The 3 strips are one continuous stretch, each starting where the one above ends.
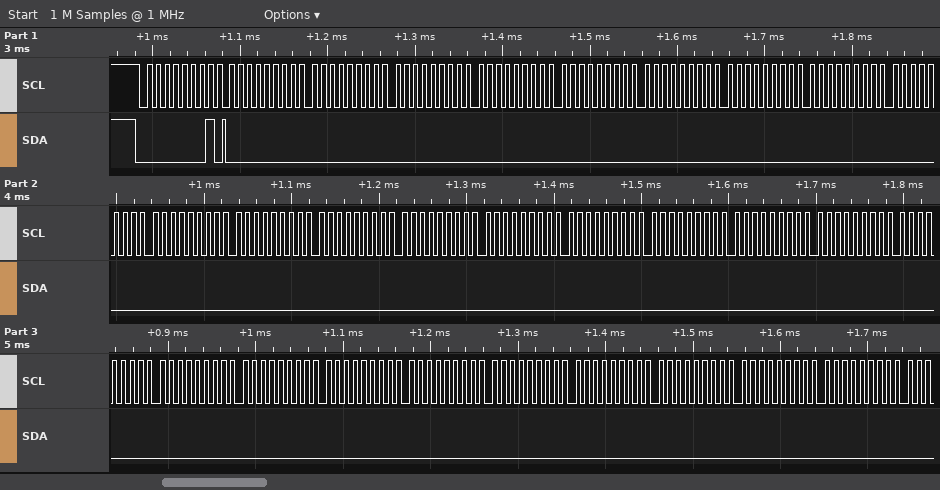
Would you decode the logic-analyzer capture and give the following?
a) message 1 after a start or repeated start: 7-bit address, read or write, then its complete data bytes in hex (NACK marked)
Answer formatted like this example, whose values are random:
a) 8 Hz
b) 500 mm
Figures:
a) 0x00 read: 00 00 00 00 00 00 00 00 00 00 00 00 00 00 00 00 00 00 00 00 00 00 00 00 00 00 00 00
